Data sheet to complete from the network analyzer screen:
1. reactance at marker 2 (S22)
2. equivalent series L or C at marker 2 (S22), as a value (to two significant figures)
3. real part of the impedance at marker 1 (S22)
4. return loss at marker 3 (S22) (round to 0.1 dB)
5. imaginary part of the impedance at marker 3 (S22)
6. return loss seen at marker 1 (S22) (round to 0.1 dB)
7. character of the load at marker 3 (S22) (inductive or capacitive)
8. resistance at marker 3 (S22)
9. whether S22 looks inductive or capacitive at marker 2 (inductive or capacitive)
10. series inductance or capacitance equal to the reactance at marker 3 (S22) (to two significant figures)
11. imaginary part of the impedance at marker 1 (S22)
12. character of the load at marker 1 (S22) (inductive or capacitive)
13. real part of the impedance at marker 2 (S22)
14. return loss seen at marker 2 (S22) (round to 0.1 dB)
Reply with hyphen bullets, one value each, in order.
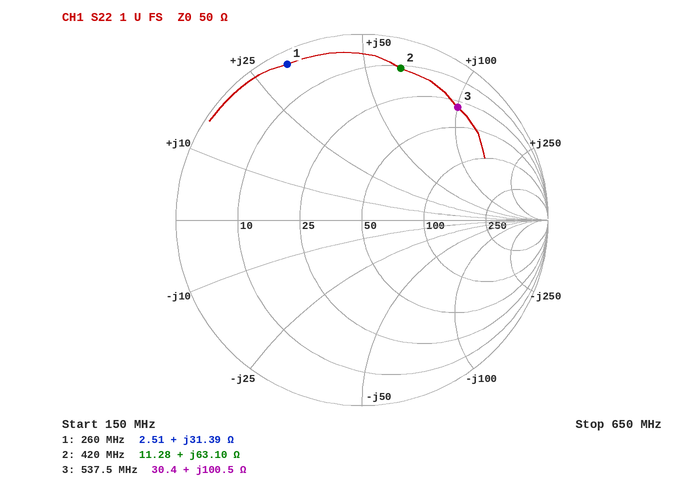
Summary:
- +63.10 Ω
- 24 nH
- 2.51 Ω
- 2.0 dB
- +100.5 Ω
- 0.6 dB
- inductive
- 30.4 Ω
- inductive
- 30 nH
- +31.39 Ω
- inductive
- 11.28 Ω
- 1.5 dB
